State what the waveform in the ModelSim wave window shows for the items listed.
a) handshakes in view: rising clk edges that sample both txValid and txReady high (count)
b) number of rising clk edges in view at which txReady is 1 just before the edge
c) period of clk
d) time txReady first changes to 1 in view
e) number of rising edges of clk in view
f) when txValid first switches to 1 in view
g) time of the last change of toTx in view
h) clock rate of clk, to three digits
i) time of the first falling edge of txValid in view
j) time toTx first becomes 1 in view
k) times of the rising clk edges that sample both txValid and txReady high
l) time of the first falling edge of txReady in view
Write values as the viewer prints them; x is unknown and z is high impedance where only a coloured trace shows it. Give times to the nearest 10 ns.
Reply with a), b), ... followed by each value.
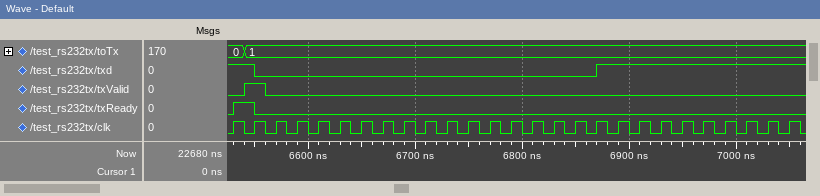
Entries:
a) 1
b) 1
c) 20 ns
d) 6530 ns
e) 27
f) 6540 ns
g) 6540 ns
h) 50.0 MHz
i) 6560 ns
j) 6540 ns
k) 6550 ns
l) 6550 ns
